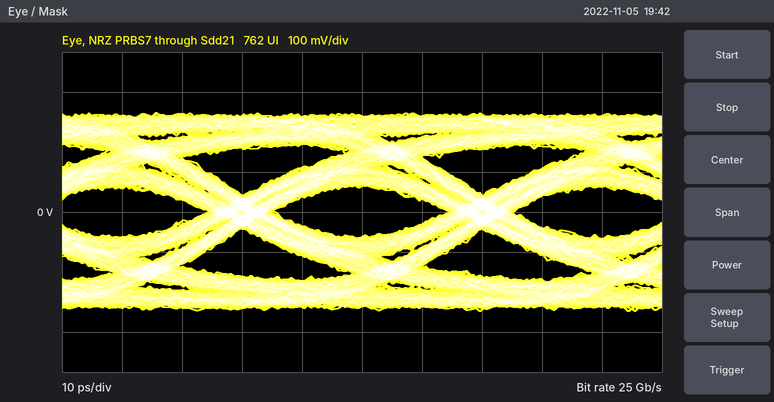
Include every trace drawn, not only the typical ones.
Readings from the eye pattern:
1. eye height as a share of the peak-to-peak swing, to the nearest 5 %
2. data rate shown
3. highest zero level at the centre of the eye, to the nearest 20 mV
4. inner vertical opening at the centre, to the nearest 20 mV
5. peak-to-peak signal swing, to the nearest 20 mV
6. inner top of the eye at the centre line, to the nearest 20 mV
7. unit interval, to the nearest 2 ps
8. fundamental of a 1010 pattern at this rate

25 %
25 Gb/s
-60 mV
120 mV
500 mV
60 mV
40 ps
12.5 GHz
